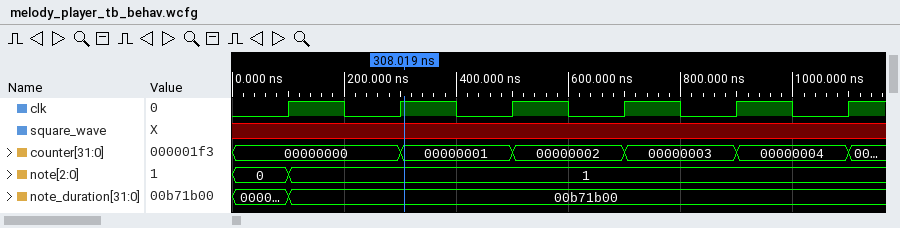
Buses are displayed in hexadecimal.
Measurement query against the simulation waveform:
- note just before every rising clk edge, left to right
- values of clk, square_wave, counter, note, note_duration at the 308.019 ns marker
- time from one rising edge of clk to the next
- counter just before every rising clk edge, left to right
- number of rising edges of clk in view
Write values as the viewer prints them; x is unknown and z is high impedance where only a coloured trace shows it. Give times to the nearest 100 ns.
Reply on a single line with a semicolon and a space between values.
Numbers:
0, 1, 1, 1, 1, 1; clk=1, square_wave=x, counter=00000001, note=1, note_duration=00b71b00; 200 ns; 00000000, 00000000, 00000001, 00000002, 00000003, 00000004; 6
